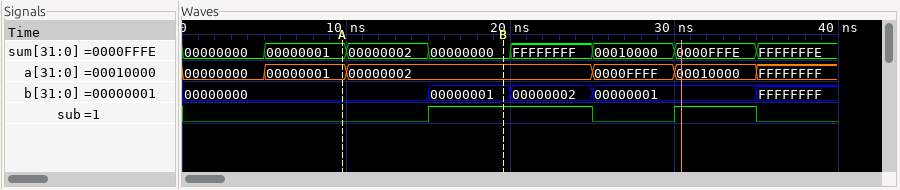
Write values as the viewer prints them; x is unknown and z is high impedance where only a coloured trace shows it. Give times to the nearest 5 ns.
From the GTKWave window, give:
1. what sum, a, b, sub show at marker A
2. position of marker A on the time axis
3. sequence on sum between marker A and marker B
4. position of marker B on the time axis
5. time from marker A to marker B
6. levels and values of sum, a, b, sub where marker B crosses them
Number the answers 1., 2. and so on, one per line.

1. sum=00000001, a=00000001, b=00000000, sub=0
2. 10 ns
3. 00000001, 00000002, 00000000
4. 20 ns
5. 10 ns
6. sum=00000000, a=00000002, b=00000001, sub=1
